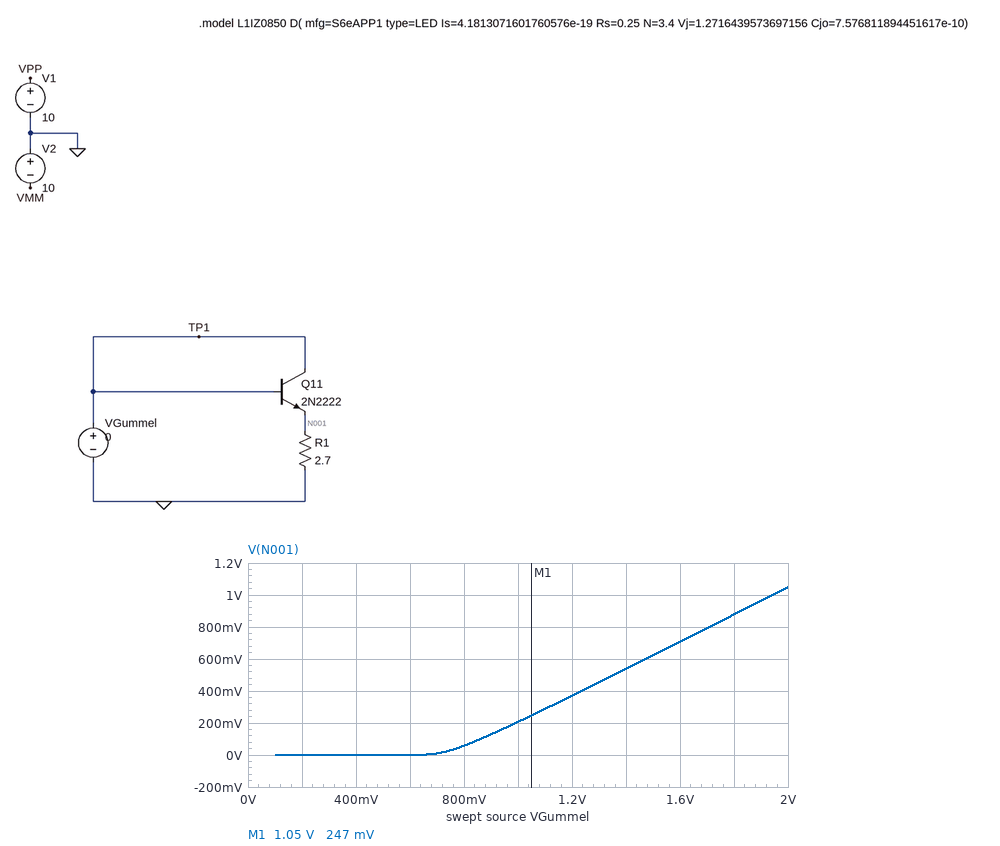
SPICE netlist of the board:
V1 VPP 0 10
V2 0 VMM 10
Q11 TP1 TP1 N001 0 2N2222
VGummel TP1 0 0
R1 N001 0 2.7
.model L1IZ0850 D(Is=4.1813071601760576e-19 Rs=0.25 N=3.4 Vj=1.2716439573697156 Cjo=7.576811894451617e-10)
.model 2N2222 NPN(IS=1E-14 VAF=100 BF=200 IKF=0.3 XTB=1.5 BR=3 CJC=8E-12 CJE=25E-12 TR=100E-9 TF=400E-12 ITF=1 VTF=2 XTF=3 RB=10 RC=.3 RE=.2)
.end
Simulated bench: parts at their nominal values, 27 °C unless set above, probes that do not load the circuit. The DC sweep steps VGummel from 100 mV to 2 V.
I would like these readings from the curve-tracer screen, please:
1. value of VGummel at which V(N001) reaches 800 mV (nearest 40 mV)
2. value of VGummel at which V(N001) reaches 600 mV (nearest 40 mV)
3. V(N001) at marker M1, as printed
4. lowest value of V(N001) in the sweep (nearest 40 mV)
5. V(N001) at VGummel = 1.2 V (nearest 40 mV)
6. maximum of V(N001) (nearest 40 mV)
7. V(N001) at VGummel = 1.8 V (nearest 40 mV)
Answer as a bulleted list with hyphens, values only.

- 1.72 V
- 1.48 V
- 247 mV
- 0 V
- 360 mV
- 1.04 V
- 880 mV
